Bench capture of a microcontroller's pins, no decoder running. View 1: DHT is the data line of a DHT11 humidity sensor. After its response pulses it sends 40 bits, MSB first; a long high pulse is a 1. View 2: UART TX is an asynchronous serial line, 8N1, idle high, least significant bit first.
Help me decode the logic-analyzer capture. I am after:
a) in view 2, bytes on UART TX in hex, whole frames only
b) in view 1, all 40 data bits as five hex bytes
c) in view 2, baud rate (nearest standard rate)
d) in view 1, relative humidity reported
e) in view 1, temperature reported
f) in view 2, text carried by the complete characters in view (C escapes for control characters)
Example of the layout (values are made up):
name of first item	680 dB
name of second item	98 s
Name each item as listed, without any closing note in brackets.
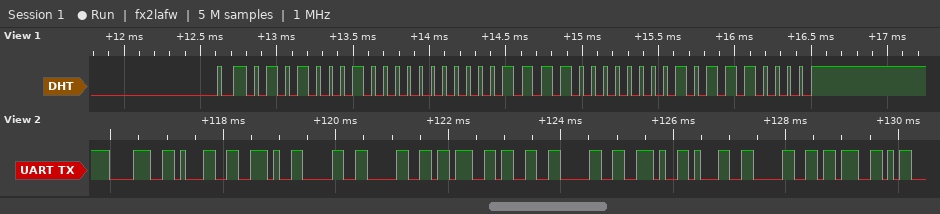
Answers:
in view 2, bytes on UART TX in hex, whole frames only	38 31 2E 30 30 3B 33 30 2E 31 30 3B
in view 1, all 40 data bits as five hex bytes	51 00 1E 01 70
in view 2, baud rate	9600 baud
in view 1, relative humidity reported	81 %
in view 1, temperature reported	30.1 °C
in view 2, text carried by the complete characters in view	"81.00;30.10;"
